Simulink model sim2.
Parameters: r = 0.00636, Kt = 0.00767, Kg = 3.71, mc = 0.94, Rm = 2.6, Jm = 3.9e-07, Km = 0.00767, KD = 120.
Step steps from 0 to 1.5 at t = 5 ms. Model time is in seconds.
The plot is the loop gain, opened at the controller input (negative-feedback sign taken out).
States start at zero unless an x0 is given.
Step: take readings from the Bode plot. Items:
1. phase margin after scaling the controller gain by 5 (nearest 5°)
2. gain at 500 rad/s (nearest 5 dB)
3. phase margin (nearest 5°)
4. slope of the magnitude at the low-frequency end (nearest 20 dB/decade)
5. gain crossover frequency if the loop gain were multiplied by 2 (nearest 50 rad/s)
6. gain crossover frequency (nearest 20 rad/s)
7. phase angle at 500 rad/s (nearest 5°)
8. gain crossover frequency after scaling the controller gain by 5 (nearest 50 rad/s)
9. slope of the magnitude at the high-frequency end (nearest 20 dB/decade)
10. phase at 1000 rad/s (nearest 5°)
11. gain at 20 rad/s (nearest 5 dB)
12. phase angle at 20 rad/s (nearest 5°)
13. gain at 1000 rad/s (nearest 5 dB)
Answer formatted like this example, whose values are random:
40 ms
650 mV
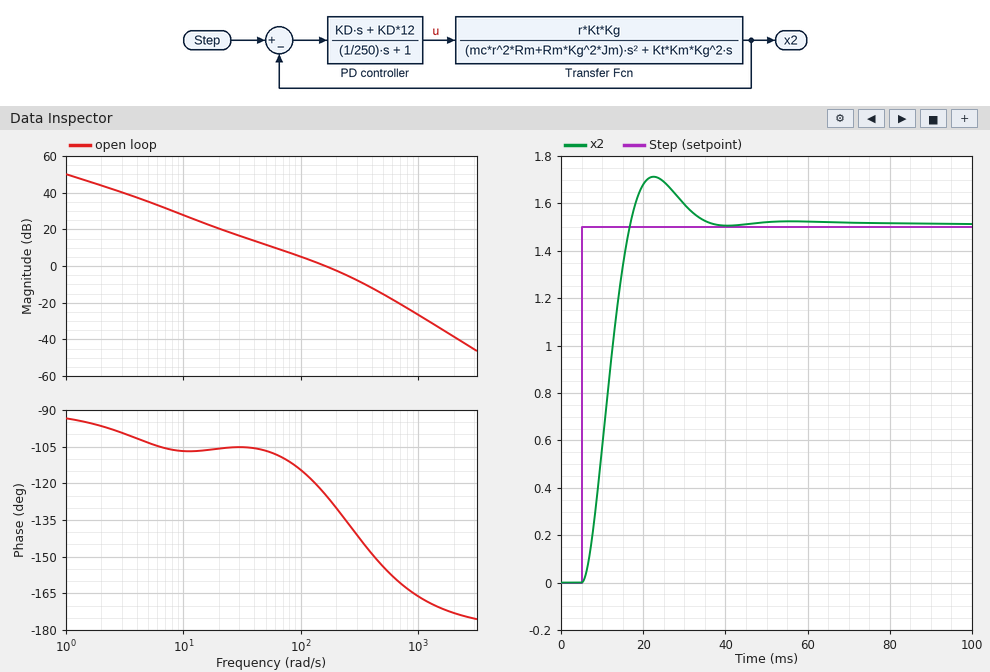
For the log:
30°
-15 dB
55°
-20 dB/decade
250 rad/s
160 rad/s
-155°
450 rad/s
-40 dB/decade
-165°
20 dB
-105°
-25 dB
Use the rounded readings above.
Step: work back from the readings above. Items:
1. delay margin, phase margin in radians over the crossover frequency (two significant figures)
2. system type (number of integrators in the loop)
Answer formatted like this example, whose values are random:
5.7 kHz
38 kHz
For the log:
0.0060 s
1
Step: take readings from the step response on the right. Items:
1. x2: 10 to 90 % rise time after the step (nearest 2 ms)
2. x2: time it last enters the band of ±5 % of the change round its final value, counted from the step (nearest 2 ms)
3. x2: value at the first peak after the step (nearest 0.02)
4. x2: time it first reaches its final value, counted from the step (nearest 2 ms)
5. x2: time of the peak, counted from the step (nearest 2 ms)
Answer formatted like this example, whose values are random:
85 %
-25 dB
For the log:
8 ms
26 ms
1.72
12 ms
18 ms
